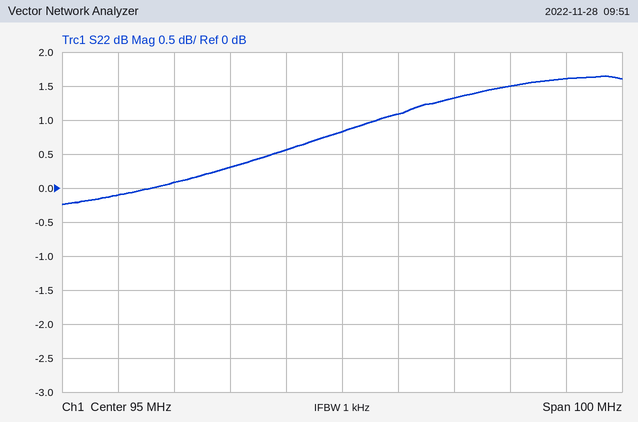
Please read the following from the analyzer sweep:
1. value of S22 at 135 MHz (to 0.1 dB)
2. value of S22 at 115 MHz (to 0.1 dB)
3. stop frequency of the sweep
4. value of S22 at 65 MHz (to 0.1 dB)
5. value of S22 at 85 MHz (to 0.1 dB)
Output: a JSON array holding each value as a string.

["1.6 dB", "1.3 dB", "145 MHz", "0.1 dB", "0.6 dB"]
